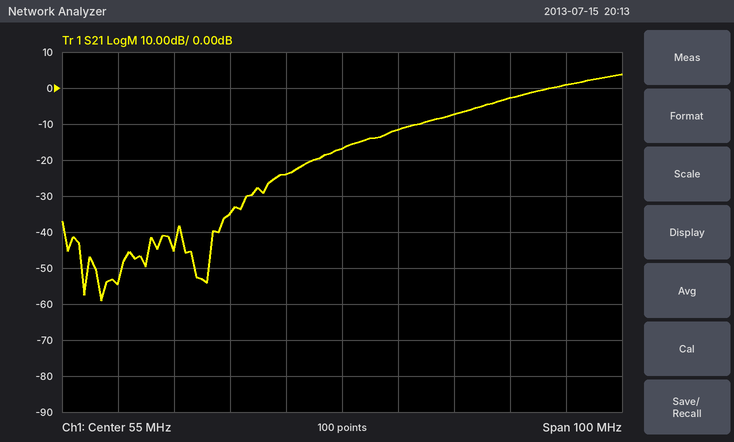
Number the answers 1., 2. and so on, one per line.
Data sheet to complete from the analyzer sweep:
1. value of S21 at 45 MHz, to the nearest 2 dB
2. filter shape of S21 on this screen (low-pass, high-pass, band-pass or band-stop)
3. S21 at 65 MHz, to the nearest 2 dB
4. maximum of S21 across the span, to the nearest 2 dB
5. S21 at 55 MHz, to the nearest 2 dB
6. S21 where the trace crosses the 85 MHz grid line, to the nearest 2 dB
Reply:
1. -24 dB
2. high-pass
3. -12 dB
4. 4 dB
5. -16 dB
6. -2 dB
